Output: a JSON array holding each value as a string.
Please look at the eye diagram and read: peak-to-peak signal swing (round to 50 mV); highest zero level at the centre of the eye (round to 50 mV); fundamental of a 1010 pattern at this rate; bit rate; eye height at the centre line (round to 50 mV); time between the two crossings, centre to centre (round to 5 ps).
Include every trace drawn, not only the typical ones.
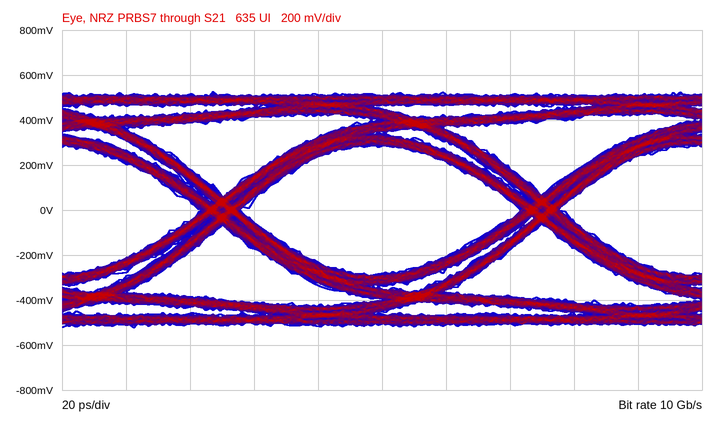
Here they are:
["1.05 V", "-300 mV", "5 GHz", "10 Gb/s", "550 mV", "100 ps"]
